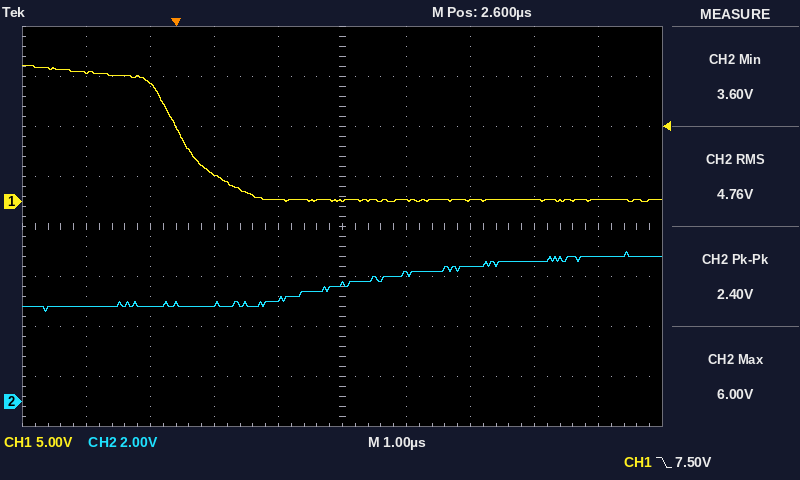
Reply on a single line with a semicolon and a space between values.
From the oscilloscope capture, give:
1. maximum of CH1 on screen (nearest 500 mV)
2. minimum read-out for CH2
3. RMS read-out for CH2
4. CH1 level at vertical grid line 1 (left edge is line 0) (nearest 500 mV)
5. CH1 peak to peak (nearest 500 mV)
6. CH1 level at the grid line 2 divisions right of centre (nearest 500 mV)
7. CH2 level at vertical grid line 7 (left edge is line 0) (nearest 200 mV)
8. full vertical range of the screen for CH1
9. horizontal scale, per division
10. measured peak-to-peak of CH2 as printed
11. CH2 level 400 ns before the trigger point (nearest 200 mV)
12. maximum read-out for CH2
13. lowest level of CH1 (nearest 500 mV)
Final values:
13.5 V; 3.60 V; 4.76 V; 13.0 V; 13.5 V; 0.0 V; 5.4 V; 40 V; 1 µs; 2.40 V; 3.8 V; 6.00 V; 0.0 V
